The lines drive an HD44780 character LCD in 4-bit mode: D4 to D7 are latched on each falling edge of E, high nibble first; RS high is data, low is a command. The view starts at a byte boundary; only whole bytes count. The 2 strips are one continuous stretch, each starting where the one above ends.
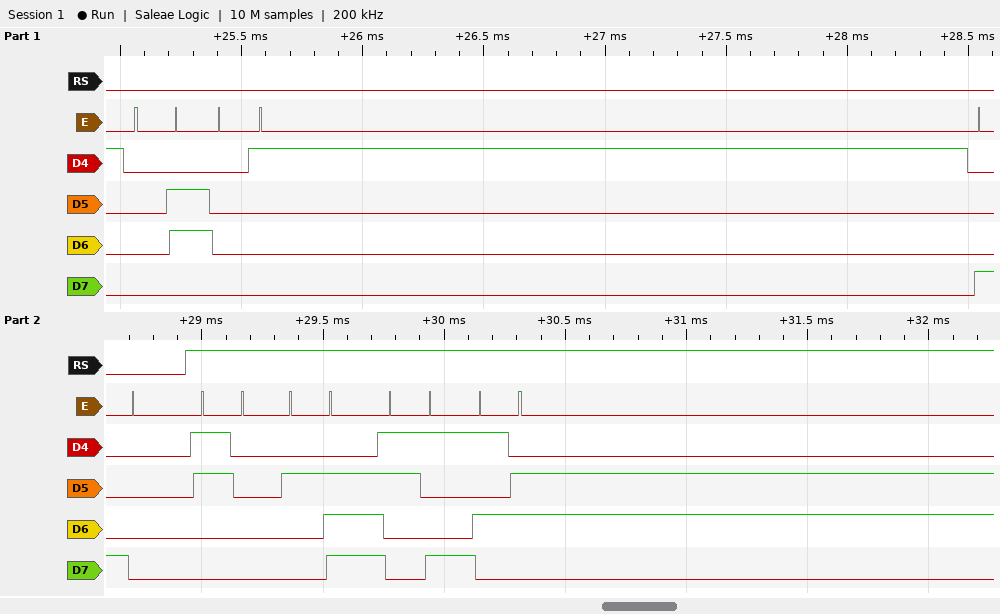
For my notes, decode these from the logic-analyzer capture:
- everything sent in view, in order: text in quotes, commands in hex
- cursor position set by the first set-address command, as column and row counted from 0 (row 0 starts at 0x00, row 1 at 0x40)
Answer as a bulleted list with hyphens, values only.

- 0x06 0x01 0x80 "0.9V"
- column 0, row 0
